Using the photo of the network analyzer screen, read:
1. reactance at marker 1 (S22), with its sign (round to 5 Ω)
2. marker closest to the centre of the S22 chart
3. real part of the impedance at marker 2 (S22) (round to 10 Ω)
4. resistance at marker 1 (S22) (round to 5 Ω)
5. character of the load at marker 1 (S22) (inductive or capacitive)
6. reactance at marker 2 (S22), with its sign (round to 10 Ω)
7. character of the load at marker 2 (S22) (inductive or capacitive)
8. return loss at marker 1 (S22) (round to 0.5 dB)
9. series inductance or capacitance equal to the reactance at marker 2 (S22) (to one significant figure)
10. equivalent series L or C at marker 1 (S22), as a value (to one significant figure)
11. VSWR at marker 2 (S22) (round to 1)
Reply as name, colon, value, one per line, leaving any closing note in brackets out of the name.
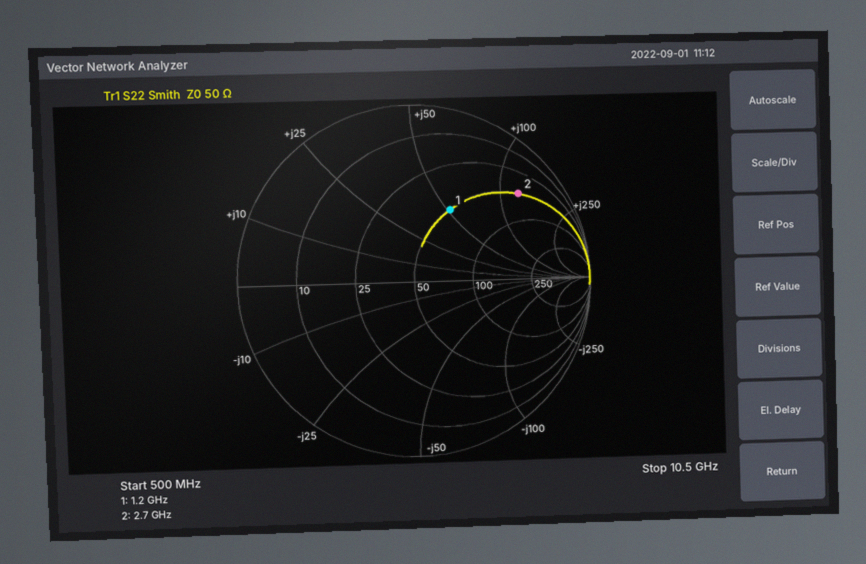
reactance at marker 1 (S22), with its sign: +50 Ω
marker closest to the centre of the S22 chart: marker 1
real part of the impedance at marker 2 (S22): 50 Ω
resistance at marker 1 (S22): 50 Ω
character of the load at marker 1 (S22): inductive
reactance at marker 2 (S22), with its sign: +120 Ω
character of the load at marker 2 (S22): inductive
return loss at marker 1 (S22): 7.0 dB
series inductance or capacitance equal to the reactance at marker 2 (S22): 7 nH
equivalent series L or C at marker 1 (S22), as a value: 7 nH
VSWR at marker 2 (S22): 8
